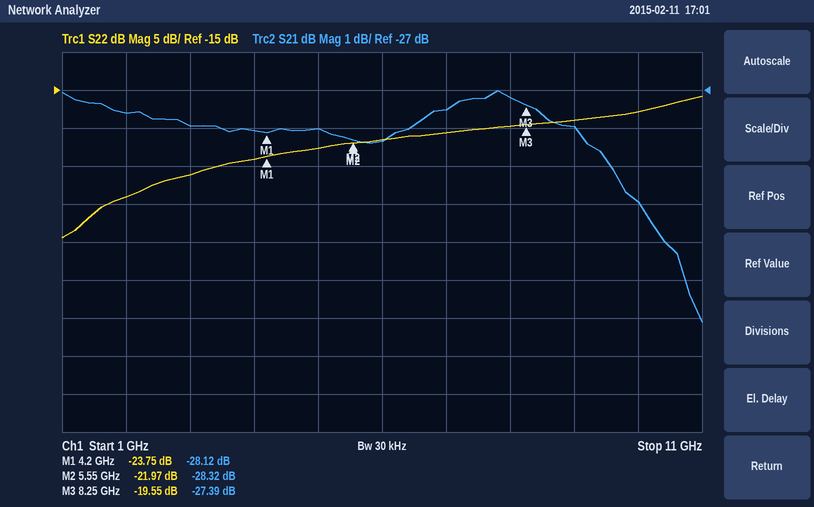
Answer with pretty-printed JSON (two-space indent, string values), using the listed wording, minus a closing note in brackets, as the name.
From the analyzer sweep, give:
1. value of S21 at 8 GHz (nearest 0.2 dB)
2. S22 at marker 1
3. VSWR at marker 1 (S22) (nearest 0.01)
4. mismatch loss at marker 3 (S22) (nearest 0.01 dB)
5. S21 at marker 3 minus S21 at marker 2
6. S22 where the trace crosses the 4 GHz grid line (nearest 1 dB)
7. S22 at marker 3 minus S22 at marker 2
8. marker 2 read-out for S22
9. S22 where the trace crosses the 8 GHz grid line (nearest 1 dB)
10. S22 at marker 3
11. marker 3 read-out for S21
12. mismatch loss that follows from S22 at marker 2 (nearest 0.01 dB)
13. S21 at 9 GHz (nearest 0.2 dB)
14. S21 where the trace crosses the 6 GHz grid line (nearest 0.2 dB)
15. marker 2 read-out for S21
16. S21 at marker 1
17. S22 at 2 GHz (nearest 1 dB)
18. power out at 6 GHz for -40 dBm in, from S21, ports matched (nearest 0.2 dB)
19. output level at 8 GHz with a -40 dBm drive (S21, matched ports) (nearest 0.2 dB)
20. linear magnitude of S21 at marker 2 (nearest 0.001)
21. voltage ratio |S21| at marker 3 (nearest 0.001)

{
  "value of S21 at 8 GHz": "-27.2 dB",
  "S22 at marker 1": "-23.75 dB",
  "VSWR at marker 1 (S22)": "1.14",
  "mismatch loss at marker 3 (S22)": "0.05 dB",
  "S21 at marker 3 minus S21 at marker 2": "0.93 dB",
  "S22 where the trace crosses the 4 GHz grid line": "-24 dB",
  "S22 at marker 3 minus S22 at marker 2": "2.42 dB",
  "marker 2 read-out for S22": "-21.97 dB",
  "S22 where the trace crosses the 8 GHz grid line": "-20 dB",
  "S22 at marker 3": "-19.55 dB",
  "marker 3 read-out for S21": "-27.39 dB",
  "mismatch loss that follows from S22 at marker 2": "0.03 dB",
  "S21 at 9 GHz": "-28.0 dB",
  "S21 where the trace crosses the 6 GHz grid line": "-28.4 dB",
  "marker 2 read-out for S21": "-28.32 dB",
  "S21 at marker 1": "-28.12 dB",
  "S22 at 2 GHz": "-29 dB",
  "power out at 6 GHz for -40 dBm in, from S21, ports matched": "-68.4 dBm",
  "output level at 8 GHz with a -40 dBm drive (S21, matched ports)": "-67.2 dBm",
  "linear magnitude of S21 at marker 2": "0.038",
  "voltage ratio |S21| at marker 3": "0.043"
}
